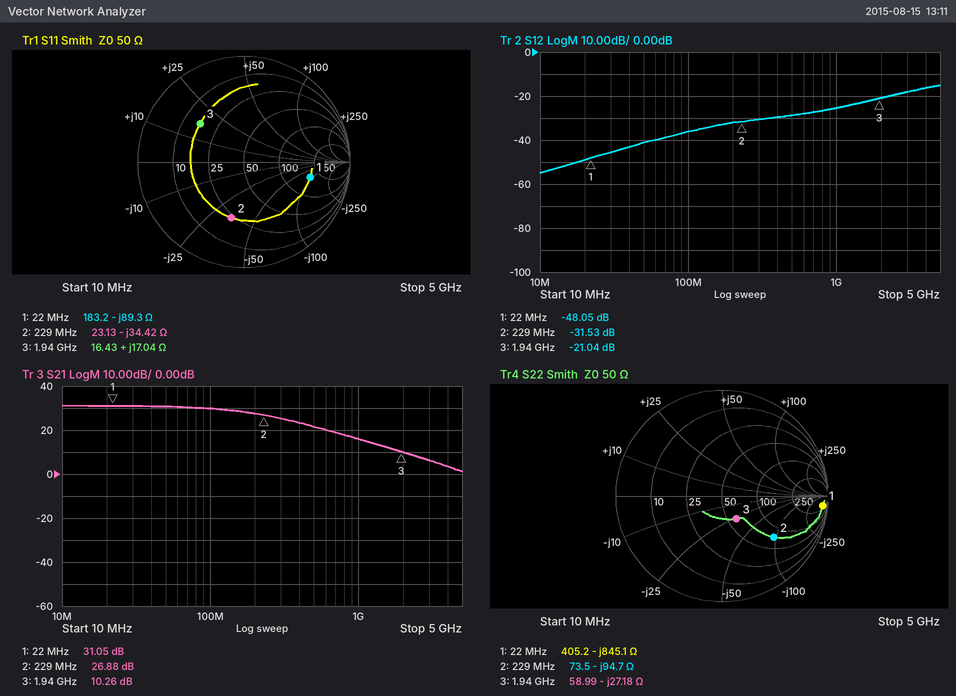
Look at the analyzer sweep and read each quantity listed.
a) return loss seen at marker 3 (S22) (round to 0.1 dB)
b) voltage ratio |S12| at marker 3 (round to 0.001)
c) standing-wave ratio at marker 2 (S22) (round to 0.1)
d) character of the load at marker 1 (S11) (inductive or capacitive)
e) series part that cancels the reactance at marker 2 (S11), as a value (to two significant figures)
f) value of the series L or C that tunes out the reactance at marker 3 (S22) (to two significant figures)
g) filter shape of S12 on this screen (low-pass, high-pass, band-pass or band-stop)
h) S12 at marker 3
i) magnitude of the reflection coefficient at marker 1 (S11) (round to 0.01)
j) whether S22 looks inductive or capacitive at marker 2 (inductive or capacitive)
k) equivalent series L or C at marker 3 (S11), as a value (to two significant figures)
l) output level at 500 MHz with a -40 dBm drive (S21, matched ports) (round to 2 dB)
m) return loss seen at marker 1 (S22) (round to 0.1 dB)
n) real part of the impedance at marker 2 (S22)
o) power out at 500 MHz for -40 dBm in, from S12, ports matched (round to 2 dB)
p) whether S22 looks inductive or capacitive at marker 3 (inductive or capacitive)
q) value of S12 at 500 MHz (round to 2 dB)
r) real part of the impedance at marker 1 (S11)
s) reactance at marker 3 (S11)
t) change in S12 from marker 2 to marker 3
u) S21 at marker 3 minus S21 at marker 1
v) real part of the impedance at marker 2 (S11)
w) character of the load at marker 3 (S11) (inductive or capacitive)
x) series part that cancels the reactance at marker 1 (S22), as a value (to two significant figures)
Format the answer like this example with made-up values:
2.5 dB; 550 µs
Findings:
11.9 dB; 0.089; 4.4; capacitive; 24 nH; 2.2 nH; high-pass; -21.04 dB; 0.64; capacitive; 1.4 nH; -18 dBm; 0.4 dB; 73.5 Ω; -68 dBm; capacitive; -28 dB; 183.2 Ω; +17.04 Ω; 10.49 dB; -20.79 dB; 23.13 Ω; inductive; 6.1 µH
